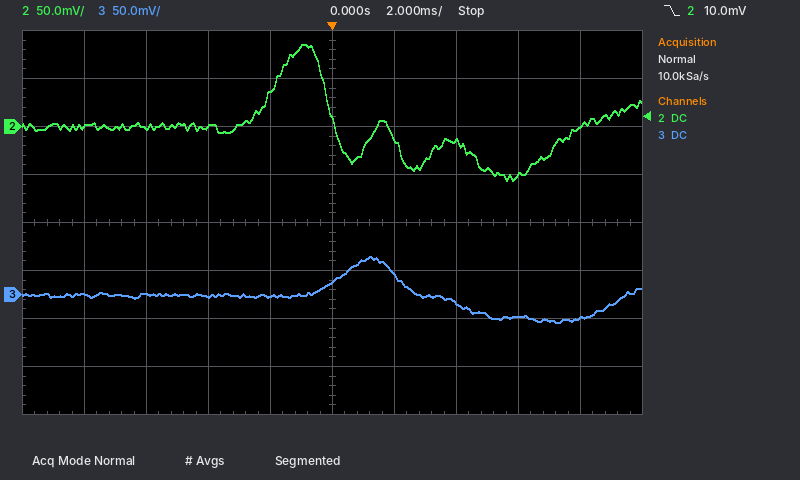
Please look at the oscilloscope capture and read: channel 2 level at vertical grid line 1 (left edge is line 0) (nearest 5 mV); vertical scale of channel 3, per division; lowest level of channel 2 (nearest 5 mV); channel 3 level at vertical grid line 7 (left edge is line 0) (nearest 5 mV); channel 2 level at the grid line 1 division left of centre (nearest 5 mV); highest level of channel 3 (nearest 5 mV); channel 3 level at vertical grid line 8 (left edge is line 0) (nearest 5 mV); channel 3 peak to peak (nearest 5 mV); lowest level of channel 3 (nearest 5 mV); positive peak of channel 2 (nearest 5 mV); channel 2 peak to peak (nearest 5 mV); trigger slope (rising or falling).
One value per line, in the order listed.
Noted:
0 mV
50 mV
-55 mV
-10 mV
35 mV
40 mV
-25 mV
70 mV
-30 mV
85 mV
140 mV
falling
